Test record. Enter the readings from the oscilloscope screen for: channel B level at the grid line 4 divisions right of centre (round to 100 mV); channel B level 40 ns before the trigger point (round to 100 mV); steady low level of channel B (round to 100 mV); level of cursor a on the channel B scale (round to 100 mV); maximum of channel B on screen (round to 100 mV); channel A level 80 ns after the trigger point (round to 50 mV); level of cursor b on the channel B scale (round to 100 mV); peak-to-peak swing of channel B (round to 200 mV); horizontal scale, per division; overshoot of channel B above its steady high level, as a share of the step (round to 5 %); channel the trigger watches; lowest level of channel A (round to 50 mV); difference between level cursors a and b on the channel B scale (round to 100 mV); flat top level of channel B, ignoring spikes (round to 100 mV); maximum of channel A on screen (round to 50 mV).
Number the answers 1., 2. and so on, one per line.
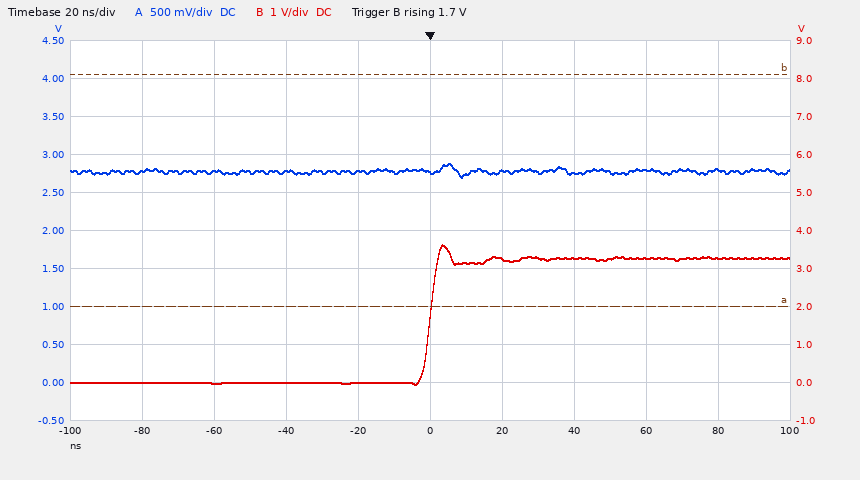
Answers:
1. 3.3 V
2. 0.0 V
3. 0.0 V
4. 2.0 V
5. 3.6 V
6. 2.80 V
7. 8.1 V
8. 3.6 V
9. 20 ns
10. 10 %
11. channel B
12. 2.70 V
13. 6.1 V
14. 3.3 V
15. 2.90 V
